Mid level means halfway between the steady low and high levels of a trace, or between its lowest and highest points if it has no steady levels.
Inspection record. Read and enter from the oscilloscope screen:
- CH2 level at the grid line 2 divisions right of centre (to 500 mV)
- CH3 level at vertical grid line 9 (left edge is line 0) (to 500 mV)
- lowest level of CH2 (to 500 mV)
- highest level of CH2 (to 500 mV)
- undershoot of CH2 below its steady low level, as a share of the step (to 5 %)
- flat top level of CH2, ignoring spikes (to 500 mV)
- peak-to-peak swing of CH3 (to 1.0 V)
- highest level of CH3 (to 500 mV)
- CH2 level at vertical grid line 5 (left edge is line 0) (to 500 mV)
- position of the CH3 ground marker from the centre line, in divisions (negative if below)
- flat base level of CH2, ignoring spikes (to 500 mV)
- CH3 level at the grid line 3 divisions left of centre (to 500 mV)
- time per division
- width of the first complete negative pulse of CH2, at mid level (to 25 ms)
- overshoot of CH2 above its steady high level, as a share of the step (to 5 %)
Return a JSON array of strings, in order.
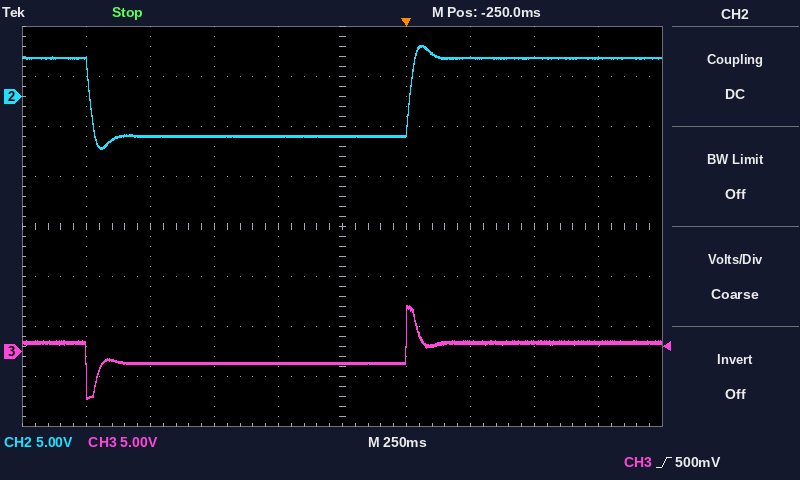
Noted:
["4.0 V", "1.0 V", "-5.0 V", "5.0 V", "15 %", "4.0 V", "9.0 V", "4.5 V", "-4.0 V", "-2.5 div", "-4.0 V", "-1.0 V", "250 ms", "1.250 s", "15 %"]
